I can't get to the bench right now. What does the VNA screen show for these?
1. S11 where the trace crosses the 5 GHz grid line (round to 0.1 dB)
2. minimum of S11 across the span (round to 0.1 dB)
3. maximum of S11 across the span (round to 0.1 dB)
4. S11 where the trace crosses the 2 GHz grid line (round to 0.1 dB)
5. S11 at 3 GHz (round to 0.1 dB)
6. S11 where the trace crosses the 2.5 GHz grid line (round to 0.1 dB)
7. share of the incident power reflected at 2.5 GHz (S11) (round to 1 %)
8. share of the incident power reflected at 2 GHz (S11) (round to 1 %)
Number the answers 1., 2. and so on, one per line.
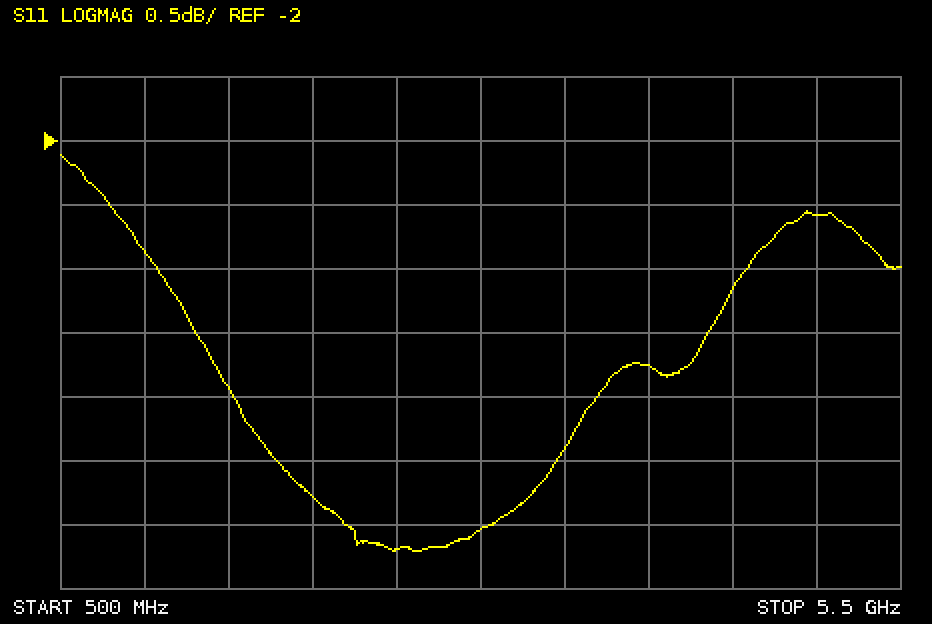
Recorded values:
1. -2.6 dB
2. -5.2 dB
3. -2.1 dB
4. -4.8 dB
5. -5.0 dB
6. -5.2 dB
7. 30 %
8. 33 %
